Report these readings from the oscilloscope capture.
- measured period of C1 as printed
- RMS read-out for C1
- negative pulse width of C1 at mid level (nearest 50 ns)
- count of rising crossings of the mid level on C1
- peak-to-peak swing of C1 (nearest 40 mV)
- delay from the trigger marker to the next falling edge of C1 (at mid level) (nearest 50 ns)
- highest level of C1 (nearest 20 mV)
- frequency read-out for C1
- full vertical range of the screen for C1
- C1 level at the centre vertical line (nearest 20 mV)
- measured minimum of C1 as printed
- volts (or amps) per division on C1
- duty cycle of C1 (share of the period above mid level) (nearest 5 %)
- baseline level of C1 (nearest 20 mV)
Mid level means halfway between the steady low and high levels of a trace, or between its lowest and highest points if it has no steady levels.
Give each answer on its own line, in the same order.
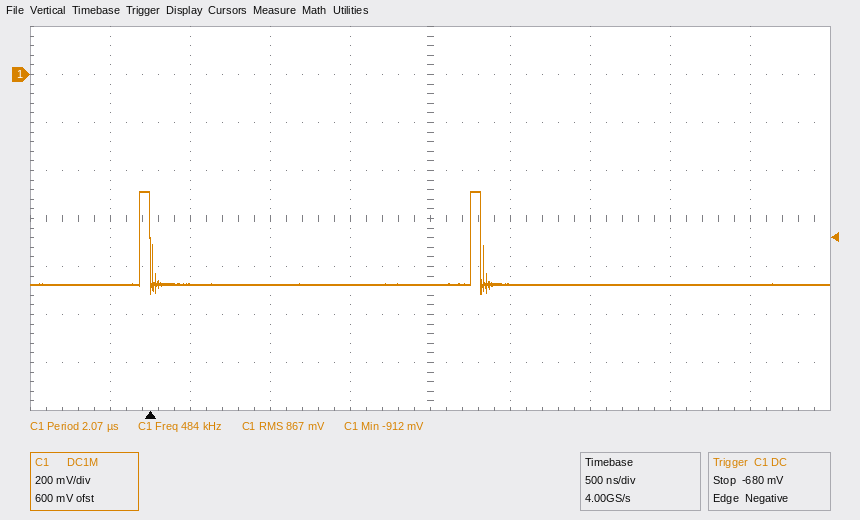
2.07 µs
867 mV
2.00 µs
2
440 mV
2.05 µs
-480 mV
484 kHz
1.6 V
-880 mV
-912 mV
200 mV
5 %
-880 mV
